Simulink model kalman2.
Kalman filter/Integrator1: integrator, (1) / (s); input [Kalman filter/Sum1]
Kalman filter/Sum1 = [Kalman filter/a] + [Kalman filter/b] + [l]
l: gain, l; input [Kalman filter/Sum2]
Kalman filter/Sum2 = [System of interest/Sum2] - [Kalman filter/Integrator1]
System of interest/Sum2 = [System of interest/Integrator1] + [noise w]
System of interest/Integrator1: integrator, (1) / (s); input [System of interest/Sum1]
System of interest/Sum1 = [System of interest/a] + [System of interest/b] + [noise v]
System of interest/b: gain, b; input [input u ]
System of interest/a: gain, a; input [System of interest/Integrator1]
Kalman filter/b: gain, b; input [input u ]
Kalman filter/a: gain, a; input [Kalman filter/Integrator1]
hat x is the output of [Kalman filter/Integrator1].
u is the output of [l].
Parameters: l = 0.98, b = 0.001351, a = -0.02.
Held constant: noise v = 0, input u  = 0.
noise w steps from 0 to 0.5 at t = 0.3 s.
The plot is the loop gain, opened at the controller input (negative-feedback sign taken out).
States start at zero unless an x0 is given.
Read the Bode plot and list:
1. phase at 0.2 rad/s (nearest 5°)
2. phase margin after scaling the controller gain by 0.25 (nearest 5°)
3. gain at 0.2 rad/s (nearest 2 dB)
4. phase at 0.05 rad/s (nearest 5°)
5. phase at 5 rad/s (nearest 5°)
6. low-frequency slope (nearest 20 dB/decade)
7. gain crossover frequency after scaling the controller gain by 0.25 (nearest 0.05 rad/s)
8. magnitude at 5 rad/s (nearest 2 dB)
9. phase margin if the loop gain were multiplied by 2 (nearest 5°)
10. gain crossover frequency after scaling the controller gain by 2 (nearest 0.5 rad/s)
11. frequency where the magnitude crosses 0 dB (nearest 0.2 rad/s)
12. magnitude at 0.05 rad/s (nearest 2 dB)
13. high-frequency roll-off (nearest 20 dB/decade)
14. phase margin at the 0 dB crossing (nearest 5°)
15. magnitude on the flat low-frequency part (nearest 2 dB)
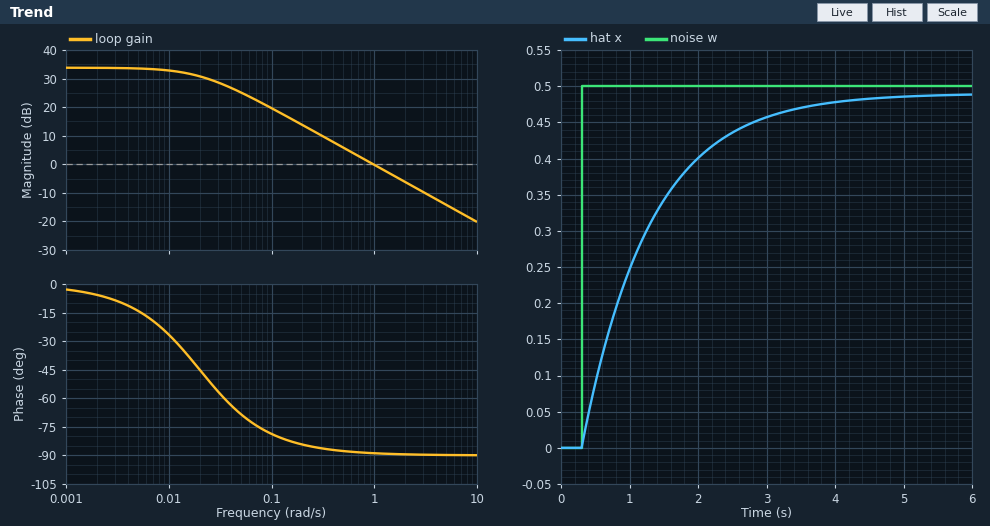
-85°
95°
14 dB
-70°
-90°
0 dB/decade
0.25 rad/s
-14 dB
90°
2.0 rad/s
1.0 rad/s
26 dB
-20 dB/decade
90°
34 dB
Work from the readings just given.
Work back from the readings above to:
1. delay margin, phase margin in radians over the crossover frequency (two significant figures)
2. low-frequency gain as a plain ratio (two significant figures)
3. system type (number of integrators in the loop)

1.6 s
50
0
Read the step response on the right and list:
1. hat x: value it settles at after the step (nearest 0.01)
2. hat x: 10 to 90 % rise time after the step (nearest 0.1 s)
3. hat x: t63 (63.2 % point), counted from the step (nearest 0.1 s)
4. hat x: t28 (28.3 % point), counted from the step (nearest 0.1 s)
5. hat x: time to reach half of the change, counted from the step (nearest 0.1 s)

0.49
2.2 s
1.0 s
0.3 s
0.7 s
